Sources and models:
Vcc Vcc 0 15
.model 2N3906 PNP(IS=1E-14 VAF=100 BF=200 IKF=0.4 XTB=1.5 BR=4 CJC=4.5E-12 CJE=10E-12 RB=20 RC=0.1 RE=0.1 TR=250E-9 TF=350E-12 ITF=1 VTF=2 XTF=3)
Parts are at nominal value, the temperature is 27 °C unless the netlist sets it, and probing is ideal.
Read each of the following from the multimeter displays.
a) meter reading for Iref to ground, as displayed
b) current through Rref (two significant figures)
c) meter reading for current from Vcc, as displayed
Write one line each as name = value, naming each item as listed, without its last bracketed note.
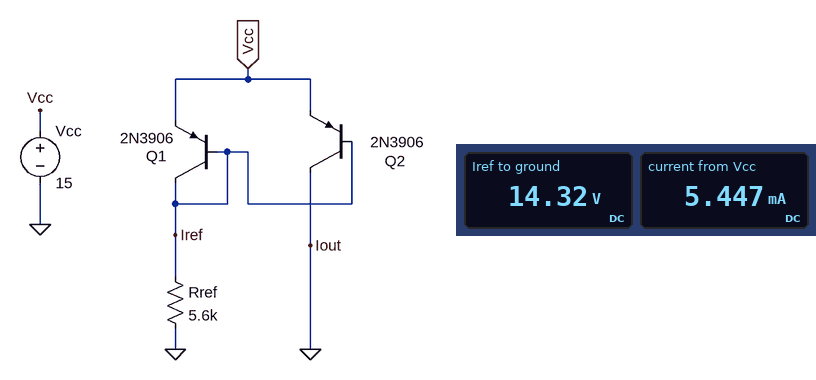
meter reading for Iref to ground, as displayed = 14.32 V
current through Rref = 2.6 mA
meter reading for current from Vcc, as displayed = 5.447 mA
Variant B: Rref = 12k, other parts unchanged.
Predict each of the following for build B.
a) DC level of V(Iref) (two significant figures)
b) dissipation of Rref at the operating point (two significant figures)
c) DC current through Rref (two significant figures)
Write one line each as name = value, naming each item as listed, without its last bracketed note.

DC level of V(Iref) = 14 V
dissipation of Rref at the operating point = 17 mW
DC current through Rref = 1.2 mA
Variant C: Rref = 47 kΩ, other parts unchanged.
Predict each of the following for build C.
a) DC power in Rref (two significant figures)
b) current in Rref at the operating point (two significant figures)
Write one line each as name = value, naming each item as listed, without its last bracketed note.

DC power in Rref = 4.4 mW
current in Rref at the operating point = 310 µA
